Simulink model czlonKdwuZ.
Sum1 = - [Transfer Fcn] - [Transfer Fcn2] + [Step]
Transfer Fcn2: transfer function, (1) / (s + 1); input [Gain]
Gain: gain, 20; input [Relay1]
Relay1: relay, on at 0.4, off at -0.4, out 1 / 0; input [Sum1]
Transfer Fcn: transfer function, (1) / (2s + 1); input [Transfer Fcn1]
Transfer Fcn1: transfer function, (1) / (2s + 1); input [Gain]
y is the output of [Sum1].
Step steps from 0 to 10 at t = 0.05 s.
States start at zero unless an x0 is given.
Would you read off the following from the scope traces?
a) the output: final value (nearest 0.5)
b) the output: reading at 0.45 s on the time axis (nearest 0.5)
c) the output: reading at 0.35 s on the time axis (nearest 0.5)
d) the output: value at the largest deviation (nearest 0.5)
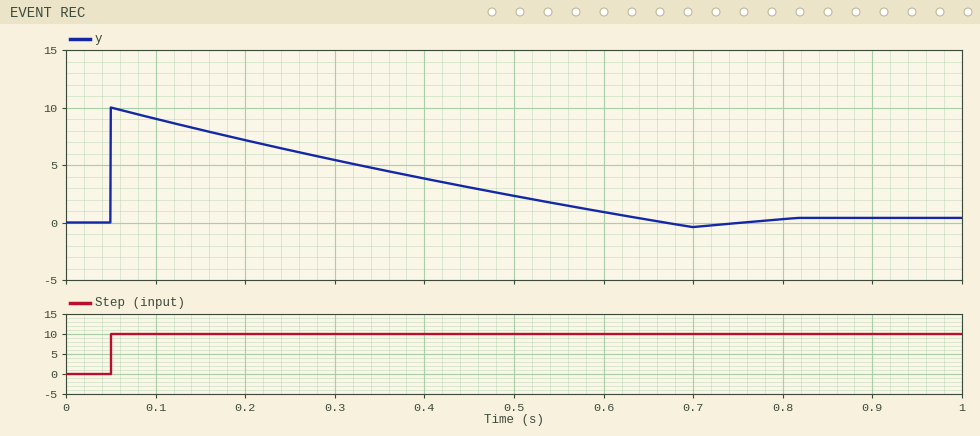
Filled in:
0.5
3.0
4.5
10.0
